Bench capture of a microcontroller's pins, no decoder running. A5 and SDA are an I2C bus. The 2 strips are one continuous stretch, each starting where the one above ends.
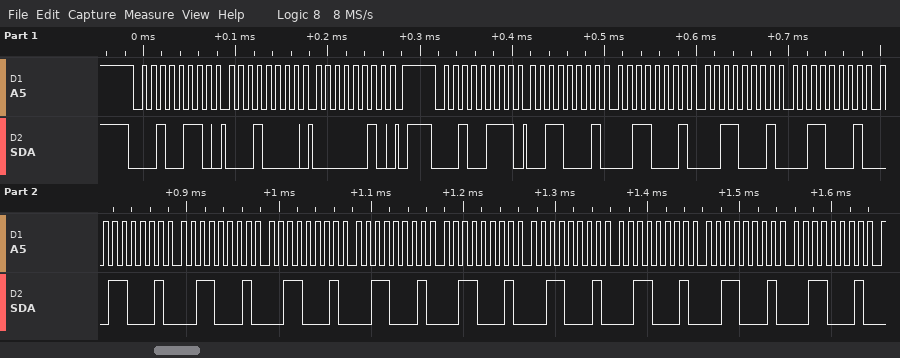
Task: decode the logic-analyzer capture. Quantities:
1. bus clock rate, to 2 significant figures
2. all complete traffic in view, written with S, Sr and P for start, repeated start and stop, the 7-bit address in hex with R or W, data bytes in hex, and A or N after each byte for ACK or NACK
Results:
100 kHz
S 13W A 10 A 02 A P S 13R A 31 A 31 A 31 A 31 A 31 A 31 A 31 A 31 A 31 A 31 A 31 A 31 A 31 A
